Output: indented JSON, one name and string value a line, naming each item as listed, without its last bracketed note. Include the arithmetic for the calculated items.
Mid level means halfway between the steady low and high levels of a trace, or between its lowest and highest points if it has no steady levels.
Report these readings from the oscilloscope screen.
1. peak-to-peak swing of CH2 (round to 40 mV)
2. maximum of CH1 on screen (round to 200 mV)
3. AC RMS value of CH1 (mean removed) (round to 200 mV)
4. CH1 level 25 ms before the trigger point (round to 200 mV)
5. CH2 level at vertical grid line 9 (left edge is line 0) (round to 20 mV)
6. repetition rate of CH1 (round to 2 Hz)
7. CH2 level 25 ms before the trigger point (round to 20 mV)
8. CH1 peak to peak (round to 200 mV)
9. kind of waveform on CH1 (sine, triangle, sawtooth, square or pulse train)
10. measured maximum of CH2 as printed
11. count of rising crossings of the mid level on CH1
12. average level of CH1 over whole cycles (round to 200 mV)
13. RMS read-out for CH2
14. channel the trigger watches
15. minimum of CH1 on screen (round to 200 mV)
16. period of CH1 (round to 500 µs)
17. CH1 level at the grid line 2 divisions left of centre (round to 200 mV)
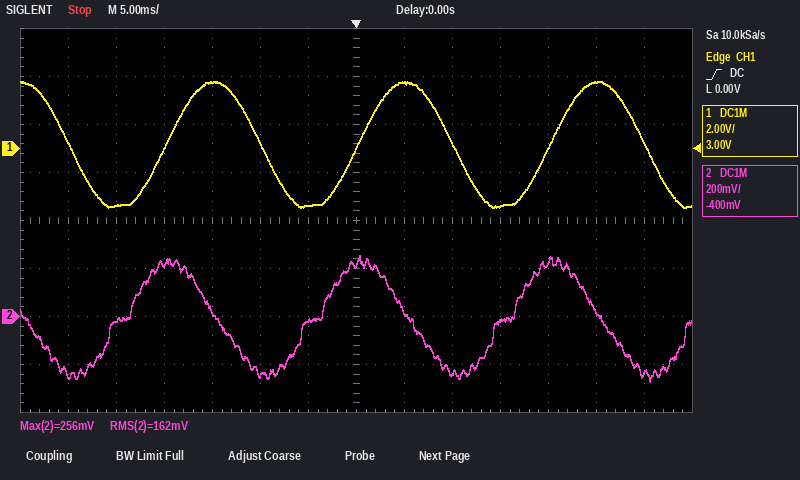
{
  "peak-to-peak swing of CH2": "520 mV",
  "maximum of CH1 on screen": "2.8 V",
  "AC RMS value of CH1 (mean removed)": "5.2 V / (2√2) ≈ 1.8 V",
  "CH1 level 25 ms before the trigger point": "-2.4 V",
  "CH2 level at vertical grid line 9 (left edge is line 0)": "-240 mV",
  "repetition rate of CH1": "1 / 20.0 ms ≈ 50 Hz",
  "CH2 level 25 ms before the trigger point": "-20 mV",
  "CH1 peak to peak": "2.8 V − (-2.4 V) = 5.2 V",
  "kind of waveform on CH1": "sine",
  "measured maximum of CH2 as printed": "256 mV",
  "count of rising crossings of the mid level on CH1": "3",
  "average level of CH1 over whole cycles": "(2.8 V + (-2.4 V)) / 2 ≈ 200 mV",
  "RMS read-out for CH2": "162 mV",
  "channel the trigger watches": "CH1",
  "minimum of CH1 on screen": "-2.4 V",
  "period of CH1": "20.0 ms",
  "CH1 level at the grid line 2 divisions left of centre": "200 mV"
}
